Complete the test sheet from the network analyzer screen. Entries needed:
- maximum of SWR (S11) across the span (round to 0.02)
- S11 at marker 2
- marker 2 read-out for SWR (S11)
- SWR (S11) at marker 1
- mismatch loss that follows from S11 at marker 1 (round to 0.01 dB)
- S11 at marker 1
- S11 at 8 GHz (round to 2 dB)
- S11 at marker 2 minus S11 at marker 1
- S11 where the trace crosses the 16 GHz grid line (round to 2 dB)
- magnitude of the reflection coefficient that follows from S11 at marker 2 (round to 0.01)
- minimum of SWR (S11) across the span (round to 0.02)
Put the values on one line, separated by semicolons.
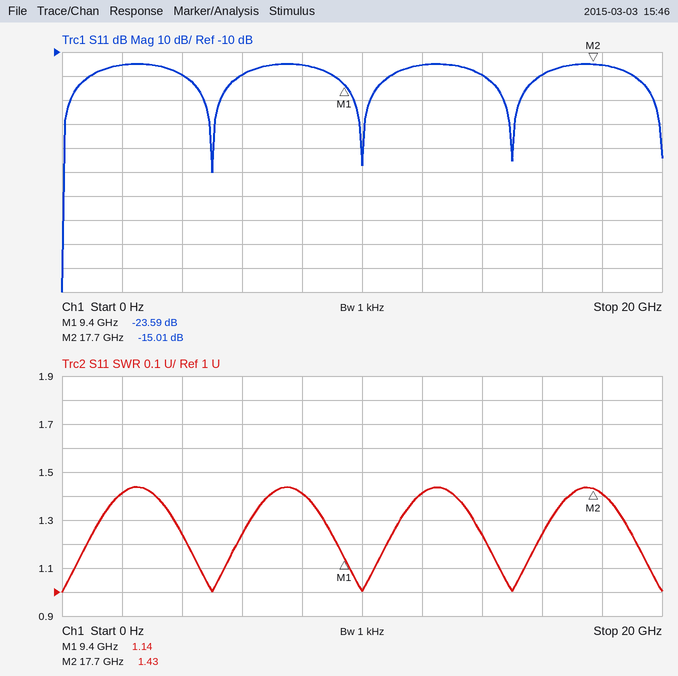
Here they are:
1.44; -15.01 dB; 1.43; 1.14; 0.02 dB; -23.59 dB; -16 dB; 8.58 dB; -20 dB; 0.18; 1.00
